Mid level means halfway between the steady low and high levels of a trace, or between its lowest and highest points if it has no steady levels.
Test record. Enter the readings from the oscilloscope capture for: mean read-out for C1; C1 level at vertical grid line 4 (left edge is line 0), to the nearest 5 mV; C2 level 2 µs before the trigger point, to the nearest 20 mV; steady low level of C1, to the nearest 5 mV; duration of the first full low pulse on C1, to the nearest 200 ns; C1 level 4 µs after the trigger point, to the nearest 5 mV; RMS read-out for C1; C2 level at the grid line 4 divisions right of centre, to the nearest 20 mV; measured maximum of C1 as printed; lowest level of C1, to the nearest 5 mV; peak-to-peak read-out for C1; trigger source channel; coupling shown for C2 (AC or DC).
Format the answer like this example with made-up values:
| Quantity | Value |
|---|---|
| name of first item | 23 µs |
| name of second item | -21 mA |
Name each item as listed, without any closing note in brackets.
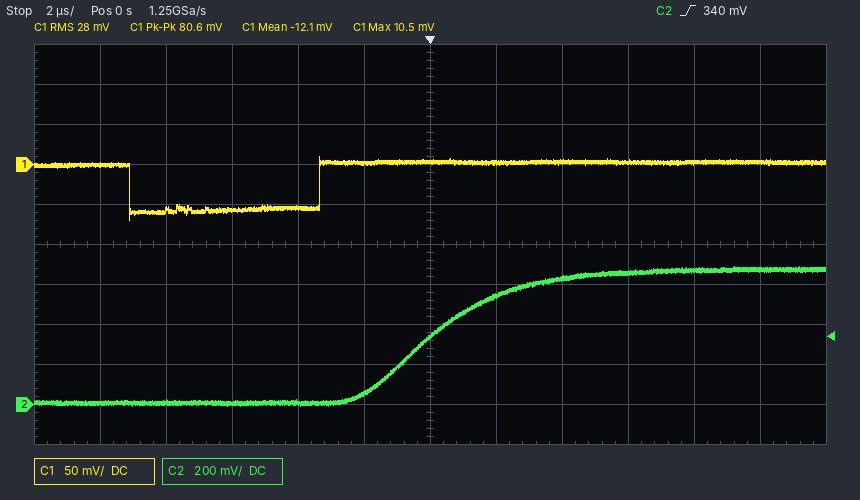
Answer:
| Quantity | Value |
|---|---|
| mean read-out for C1 | -12.1 mV |
| C1 level at vertical grid line 4 (left edge is line 0), to the nearest 5 mV | -55 mV |
| C2 level 2 µs before the trigger point, to the nearest 20 mV | 60 mV |
| steady low level of C1, to the nearest 5 mV | -55 mV |
| duration of the first full low pulse on C1, to the nearest 200 ns | 5.8 µs |
| C1 level 4 µs after the trigger point, to the nearest 5 mV | 5 mV |
| RMS read-out for C1 | 28 mV |
| C2 level at the grid line 4 divisions right of centre, to the nearest 20 mV | 660 mV |
| measured maximum of C1 as printed | 10.5 mV |
| lowest level of C1, to the nearest 5 mV | -70 mV |
| peak-to-peak read-out for C1 | 80.6 mV |
| trigger source channel | C2 |
| coupling shown for C2 | DC |
